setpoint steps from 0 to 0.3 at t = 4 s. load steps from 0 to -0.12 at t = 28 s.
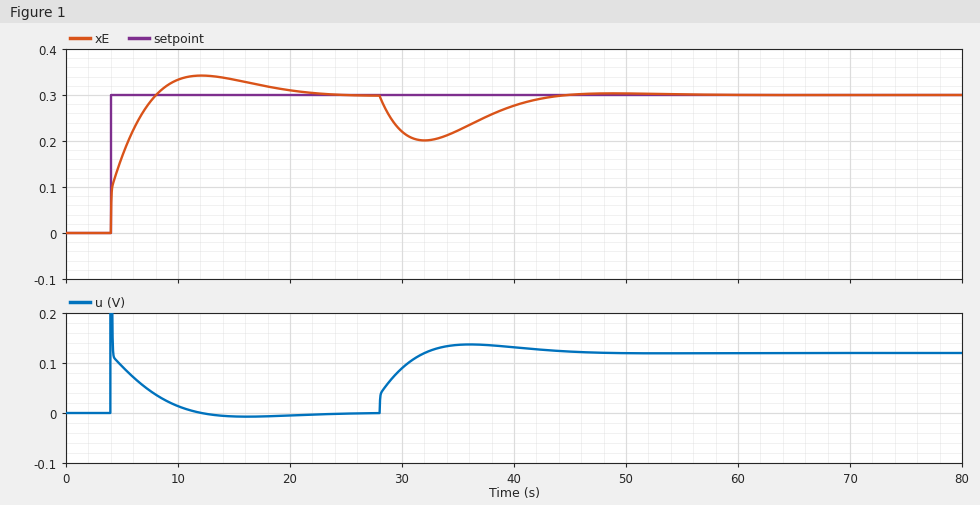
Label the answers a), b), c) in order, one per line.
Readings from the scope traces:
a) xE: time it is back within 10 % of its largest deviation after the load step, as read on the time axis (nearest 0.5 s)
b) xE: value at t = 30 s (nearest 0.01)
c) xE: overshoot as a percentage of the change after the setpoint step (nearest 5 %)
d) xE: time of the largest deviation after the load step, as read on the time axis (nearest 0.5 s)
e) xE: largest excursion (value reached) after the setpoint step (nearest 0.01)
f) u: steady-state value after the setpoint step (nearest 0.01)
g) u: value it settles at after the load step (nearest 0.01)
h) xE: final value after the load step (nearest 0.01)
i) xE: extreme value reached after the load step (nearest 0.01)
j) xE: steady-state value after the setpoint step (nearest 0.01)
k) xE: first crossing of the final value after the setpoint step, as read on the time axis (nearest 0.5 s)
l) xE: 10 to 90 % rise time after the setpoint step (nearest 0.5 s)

a) 42.0 s
b) 0.22
c) 15 %
d) 32.0 s
e) 0.34
f) 0.00
g) 0.12
h) 0.30
i) 0.20
j) 0.30
k) 8.0 s
l) 3.0 s
